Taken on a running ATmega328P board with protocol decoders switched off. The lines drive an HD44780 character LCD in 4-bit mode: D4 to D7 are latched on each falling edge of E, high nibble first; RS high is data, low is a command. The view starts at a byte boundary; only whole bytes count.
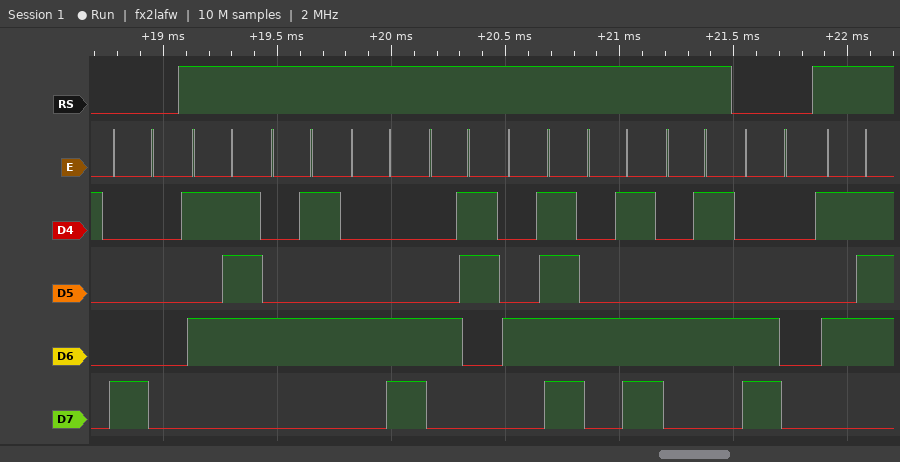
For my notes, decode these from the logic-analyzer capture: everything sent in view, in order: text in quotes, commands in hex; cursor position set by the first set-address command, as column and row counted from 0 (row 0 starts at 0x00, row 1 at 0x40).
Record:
0x80 "WELCOME" 0xC0 "W"
column 0, row 0
